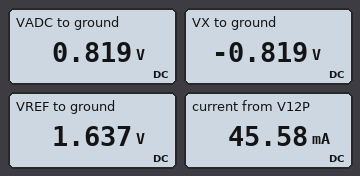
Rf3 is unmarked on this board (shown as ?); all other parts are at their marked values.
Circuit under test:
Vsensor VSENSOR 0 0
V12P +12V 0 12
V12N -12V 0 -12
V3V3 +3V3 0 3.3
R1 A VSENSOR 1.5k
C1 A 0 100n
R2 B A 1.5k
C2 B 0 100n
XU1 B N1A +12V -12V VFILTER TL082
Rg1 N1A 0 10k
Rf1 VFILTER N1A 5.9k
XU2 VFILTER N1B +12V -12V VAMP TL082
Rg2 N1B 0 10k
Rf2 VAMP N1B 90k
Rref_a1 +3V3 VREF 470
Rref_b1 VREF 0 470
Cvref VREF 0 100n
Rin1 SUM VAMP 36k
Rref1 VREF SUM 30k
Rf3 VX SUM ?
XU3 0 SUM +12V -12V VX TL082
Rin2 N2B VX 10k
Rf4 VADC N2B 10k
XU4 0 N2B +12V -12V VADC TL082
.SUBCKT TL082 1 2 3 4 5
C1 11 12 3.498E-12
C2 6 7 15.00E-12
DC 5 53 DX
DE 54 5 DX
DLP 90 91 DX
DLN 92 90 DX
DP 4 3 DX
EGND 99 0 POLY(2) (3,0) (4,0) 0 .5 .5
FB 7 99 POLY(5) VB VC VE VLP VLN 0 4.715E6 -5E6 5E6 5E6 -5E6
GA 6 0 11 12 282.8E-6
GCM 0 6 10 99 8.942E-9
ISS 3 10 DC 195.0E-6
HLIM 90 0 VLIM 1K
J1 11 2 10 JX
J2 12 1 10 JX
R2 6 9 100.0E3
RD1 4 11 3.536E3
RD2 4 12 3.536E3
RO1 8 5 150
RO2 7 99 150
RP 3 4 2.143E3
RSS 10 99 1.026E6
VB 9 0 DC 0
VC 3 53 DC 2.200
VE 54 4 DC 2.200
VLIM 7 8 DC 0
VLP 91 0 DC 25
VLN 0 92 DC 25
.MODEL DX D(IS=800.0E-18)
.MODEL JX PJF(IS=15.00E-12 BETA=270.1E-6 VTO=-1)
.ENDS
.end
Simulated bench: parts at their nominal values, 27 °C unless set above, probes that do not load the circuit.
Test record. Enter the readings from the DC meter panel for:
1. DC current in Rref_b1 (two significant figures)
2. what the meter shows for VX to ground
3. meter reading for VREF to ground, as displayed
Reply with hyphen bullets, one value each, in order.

- 3.5 mA
- -0.819 V
- 1.637 V
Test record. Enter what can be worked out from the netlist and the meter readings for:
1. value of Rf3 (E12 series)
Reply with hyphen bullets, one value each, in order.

- 15 kΩ
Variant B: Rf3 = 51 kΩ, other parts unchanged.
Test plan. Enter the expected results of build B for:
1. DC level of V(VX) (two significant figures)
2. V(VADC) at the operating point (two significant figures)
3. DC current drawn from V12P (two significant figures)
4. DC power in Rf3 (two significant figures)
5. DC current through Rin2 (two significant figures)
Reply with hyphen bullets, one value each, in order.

- -2.8 V
- 2.8 V
- 46 mA
- 150 µW
- 280 µA
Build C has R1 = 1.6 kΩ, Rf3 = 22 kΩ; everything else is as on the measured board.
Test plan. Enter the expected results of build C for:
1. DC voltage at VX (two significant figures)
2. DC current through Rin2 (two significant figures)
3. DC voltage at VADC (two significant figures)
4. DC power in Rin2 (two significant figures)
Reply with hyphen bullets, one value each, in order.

- -1.2 V
- 120 µA
- 1.2 V
- 140 µW
